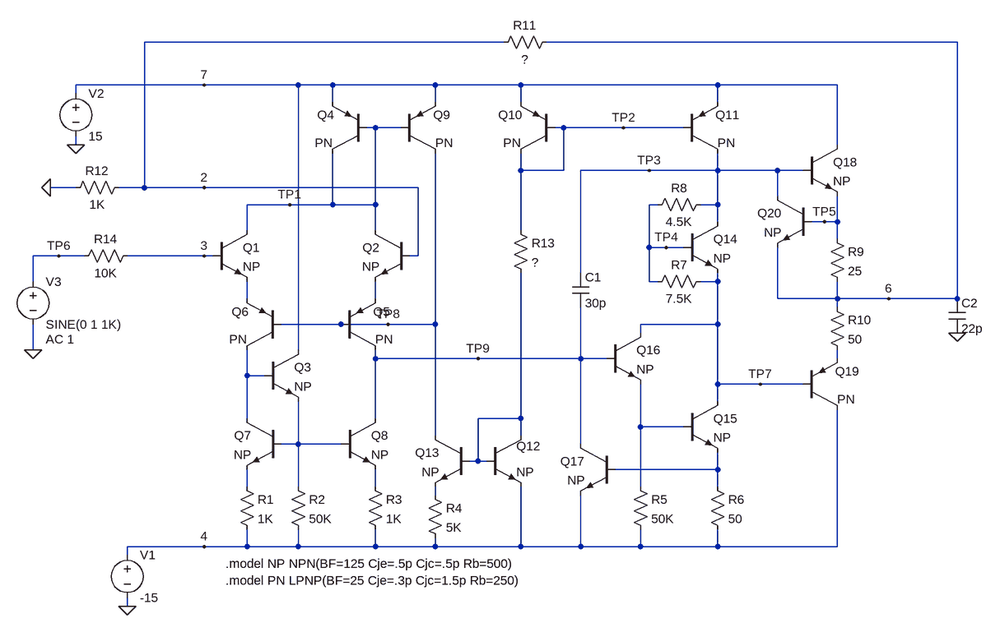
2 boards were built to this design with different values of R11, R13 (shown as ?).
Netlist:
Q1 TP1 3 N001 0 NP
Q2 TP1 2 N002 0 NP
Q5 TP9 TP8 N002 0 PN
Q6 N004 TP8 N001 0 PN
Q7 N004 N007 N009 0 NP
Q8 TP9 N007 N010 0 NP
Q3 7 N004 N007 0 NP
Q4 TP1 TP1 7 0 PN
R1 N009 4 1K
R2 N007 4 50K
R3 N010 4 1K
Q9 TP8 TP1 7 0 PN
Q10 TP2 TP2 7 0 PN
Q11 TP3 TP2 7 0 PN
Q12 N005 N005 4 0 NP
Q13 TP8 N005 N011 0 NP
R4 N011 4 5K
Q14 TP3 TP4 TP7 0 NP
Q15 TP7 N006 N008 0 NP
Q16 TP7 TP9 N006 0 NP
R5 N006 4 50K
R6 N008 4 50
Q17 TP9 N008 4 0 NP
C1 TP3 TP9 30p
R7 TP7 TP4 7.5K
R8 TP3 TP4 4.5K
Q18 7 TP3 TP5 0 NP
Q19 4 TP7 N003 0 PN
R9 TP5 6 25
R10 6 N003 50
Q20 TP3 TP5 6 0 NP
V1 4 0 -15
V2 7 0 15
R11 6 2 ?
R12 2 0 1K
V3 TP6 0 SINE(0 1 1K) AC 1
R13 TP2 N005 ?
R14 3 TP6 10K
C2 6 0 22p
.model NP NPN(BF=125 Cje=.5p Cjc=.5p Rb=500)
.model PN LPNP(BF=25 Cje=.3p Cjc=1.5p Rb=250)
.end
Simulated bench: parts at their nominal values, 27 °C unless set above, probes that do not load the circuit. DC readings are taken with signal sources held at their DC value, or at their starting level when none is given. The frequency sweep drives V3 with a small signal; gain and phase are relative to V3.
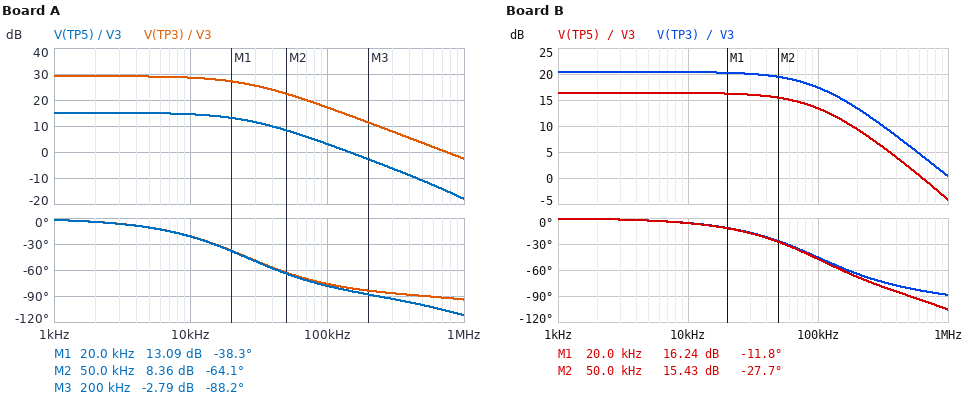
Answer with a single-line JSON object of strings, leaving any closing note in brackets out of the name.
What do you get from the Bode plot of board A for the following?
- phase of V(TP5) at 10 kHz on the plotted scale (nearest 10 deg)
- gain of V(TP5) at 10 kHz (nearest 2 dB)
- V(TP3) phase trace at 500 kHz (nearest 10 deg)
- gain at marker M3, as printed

{"phase of V(TP5) at 10 kHz on the plotted scale": "-20 deg", "gain of V(TP5) at 10 kHz": "14 dB", "V(TP3) phase trace at 500 kHz": "-90 deg", "gain at marker M3, as printed": "-2.79 dB"}
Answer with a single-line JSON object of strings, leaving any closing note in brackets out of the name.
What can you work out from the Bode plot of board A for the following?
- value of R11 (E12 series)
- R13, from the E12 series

{"value of R11": "4.7 kΩ", "R13, from the E12 series": "120 kΩ"}
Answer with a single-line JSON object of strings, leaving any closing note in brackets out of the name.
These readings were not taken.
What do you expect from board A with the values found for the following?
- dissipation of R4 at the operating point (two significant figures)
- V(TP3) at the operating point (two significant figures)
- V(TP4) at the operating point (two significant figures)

{"dissipation of R4 at the operating point": "1.1 µW", "V(TP3) at the operating point": "570 mV", "V(TP4) at the operating point": "130 mV"}
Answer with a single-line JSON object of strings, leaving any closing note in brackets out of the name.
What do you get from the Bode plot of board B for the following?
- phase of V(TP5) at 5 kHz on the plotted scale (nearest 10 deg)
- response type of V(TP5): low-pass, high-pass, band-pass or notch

{"phase of V(TP5) at 5 kHz on the plotted scale": "0 deg", "response type of V(TP5): low-pass, high-pass, band-pass or notch": "low-pass"}
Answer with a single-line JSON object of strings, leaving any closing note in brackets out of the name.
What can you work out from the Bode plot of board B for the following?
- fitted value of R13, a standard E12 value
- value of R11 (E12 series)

{"fitted value of R13, a standard E12 value": "33 kΩ", "value of R11": "5.6 kΩ"}
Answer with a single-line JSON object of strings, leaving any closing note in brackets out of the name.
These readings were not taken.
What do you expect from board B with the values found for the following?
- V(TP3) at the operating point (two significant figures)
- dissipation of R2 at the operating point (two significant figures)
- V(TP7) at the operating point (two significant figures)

{"V(TP3) at the operating point": "620 mV", "dissipation of R2 at the operating point": "8.8 µW", "V(TP7) at the operating point": "-630 mV"}
